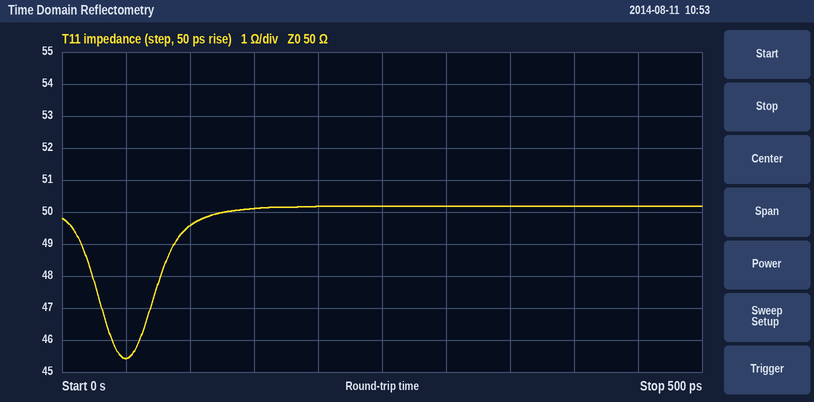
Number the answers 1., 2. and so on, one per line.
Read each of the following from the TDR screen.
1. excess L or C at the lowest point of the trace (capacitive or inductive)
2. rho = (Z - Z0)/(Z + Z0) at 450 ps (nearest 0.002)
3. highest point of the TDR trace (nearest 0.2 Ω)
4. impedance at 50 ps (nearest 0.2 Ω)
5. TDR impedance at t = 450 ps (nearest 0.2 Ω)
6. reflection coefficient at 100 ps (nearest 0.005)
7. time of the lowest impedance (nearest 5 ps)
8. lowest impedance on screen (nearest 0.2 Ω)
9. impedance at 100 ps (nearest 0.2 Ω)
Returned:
1. capacitive
2. +0.002
3. 50.2 Ω
4. 45.4 Ω
5. 50.2 Ω
6. -0.005
7. 50 ps
8. 45.4 Ω
9. 49.6 Ω
